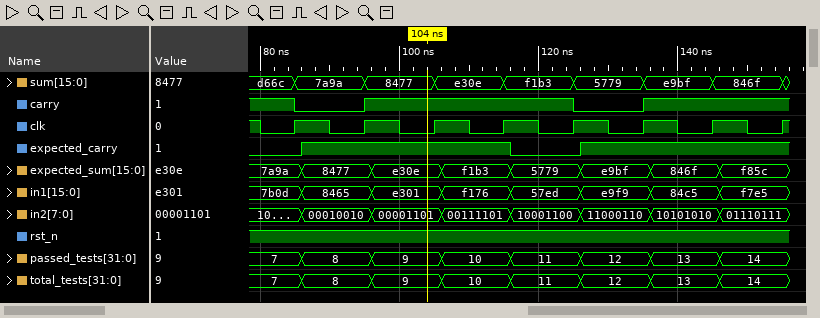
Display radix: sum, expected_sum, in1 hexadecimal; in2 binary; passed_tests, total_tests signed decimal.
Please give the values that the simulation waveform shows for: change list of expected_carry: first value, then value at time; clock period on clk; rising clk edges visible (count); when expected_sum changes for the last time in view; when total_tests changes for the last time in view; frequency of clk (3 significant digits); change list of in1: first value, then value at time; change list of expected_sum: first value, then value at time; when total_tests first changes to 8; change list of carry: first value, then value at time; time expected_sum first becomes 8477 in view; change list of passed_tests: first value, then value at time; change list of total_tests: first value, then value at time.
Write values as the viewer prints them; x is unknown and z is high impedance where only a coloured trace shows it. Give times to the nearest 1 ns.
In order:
0, 1 at 86 ns, 0 at 116 ns, 1 at 126 ns
10 ns
8
146 ns
146 ns
100 MHz
7b0d, 8465 at 86 ns, e301 at 96 ns, f176 at 106 ns, 57ed at 116 ns, e9f9 at 126 ns, 84c5 at 136 ns, f7e5 at 146 ns
7a9a, 8477 at 86 ns, e30e at 96 ns, f1b3 at 106 ns, 5779 at 116 ns, e9bf at 126 ns, 846f at 136 ns, f85c at 146 ns
86 ns
1, 0 at 85 ns, 1 at 95 ns, 0 at 125 ns, 1 at 135 ns
86 ns
7, 8 at 86 ns, 9 at 96 ns, 10 at 106 ns, 11 at 116 ns, 12 at 126 ns, 13 at 136 ns, 14 at 146 ns
7, 8 at 86 ns, 9 at 96 ns, 10 at 106 ns, 11 at 116 ns, 12 at 126 ns, 13 at 136 ns, 14 at 146 ns
